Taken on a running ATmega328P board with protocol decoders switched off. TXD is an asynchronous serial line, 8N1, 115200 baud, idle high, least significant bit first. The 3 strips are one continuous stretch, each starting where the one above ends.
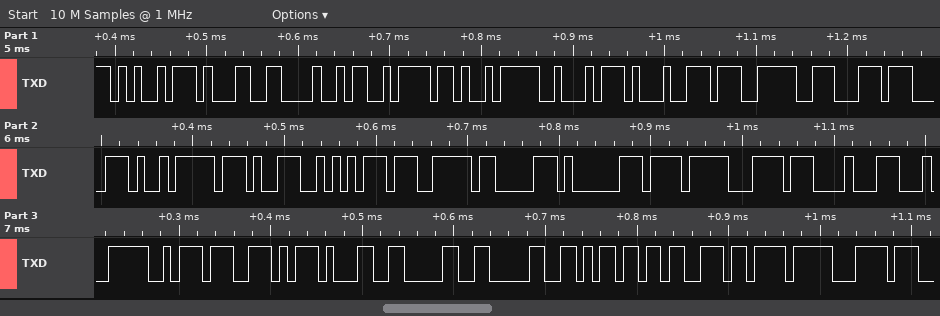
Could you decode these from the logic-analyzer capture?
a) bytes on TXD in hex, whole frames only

A5 31 48 7A E9 A2 91 E7 8E 87 E9 97 AA E7 83 81 EF BC 88 E4 BA AE 31 30 30 6D 73 EF BC
